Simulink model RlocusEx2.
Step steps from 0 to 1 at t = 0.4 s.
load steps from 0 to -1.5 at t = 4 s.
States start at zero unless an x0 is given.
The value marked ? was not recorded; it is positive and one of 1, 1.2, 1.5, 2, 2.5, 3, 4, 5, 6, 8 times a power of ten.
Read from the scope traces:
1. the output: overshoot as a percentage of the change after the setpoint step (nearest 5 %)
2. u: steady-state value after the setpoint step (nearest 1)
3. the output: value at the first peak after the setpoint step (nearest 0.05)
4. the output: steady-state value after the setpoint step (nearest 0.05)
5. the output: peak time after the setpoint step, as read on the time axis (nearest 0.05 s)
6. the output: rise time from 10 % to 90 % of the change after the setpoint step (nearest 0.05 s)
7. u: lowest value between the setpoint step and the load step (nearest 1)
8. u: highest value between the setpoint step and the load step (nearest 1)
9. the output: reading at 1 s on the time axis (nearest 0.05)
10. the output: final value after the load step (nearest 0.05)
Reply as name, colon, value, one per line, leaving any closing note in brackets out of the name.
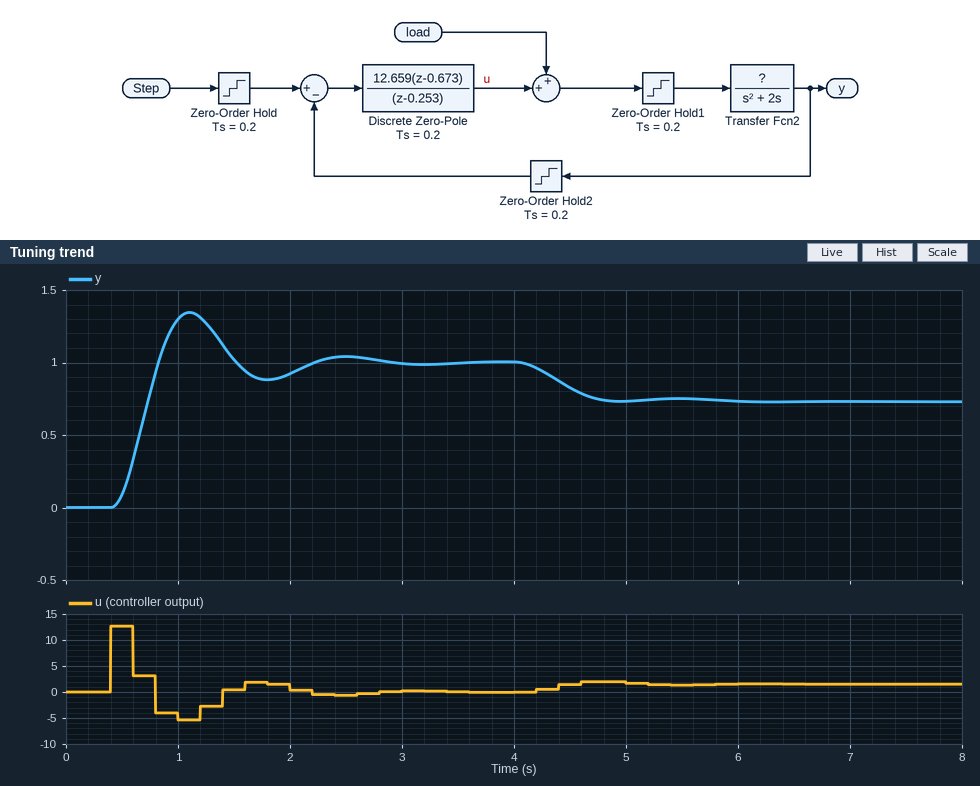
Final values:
the output: overshoot as a percentage of the change after the setpoint step: 35 %
u: steady-state value after the setpoint step: 0
the output: value at the first peak after the setpoint step: 1.35
the output: steady-state value after the setpoint step: 1.00
the output: peak time after the setpoint step, as read on the time axis: 1.10 s
the output: rise time from 10 % to 90 % of the change after the setpoint step: 0.30 s
u: lowest value between the setpoint step and the load step: -5
u: highest value between the setpoint step and the load step: 13
the output: reading at 1 s on the time axis: 1.30
the output: final value after the load step: 0.75
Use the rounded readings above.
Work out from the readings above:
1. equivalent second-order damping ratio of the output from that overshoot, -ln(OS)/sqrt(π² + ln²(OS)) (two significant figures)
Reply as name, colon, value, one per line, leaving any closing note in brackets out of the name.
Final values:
equivalent second-order damping ratio of the output from that overshoot, -ln(OS)/sqrt(π² + ln²(OS)): 0.32
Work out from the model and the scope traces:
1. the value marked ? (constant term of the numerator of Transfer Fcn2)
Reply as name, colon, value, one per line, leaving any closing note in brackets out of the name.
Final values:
the value marked ?: 1.5
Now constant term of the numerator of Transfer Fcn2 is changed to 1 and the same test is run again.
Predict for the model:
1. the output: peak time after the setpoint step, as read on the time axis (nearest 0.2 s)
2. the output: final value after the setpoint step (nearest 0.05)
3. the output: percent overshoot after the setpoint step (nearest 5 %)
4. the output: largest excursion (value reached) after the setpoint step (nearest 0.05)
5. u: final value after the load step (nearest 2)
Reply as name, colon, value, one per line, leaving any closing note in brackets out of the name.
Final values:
the output: peak time after the setpoint step, as read on the time axis: 1.4 s
the output: final value after the setpoint step: 1.00
the output: percent overshoot after the setpoint step: 15 %
the output: largest excursion (value reached) after the setpoint step: 1.15
u: final value after the load step: 2
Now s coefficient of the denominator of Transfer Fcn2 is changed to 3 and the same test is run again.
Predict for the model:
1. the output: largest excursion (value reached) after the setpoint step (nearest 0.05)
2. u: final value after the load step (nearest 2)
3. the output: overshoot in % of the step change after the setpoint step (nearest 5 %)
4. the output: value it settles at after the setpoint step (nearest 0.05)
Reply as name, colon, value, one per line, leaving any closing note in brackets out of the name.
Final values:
the output: largest excursion (value reached) after the setpoint step: 1.15
u: final value after the load step: 2
the output: overshoot in % of the step change after the setpoint step: 15 %
the output: value it settles at after the setpoint step: 1.00
